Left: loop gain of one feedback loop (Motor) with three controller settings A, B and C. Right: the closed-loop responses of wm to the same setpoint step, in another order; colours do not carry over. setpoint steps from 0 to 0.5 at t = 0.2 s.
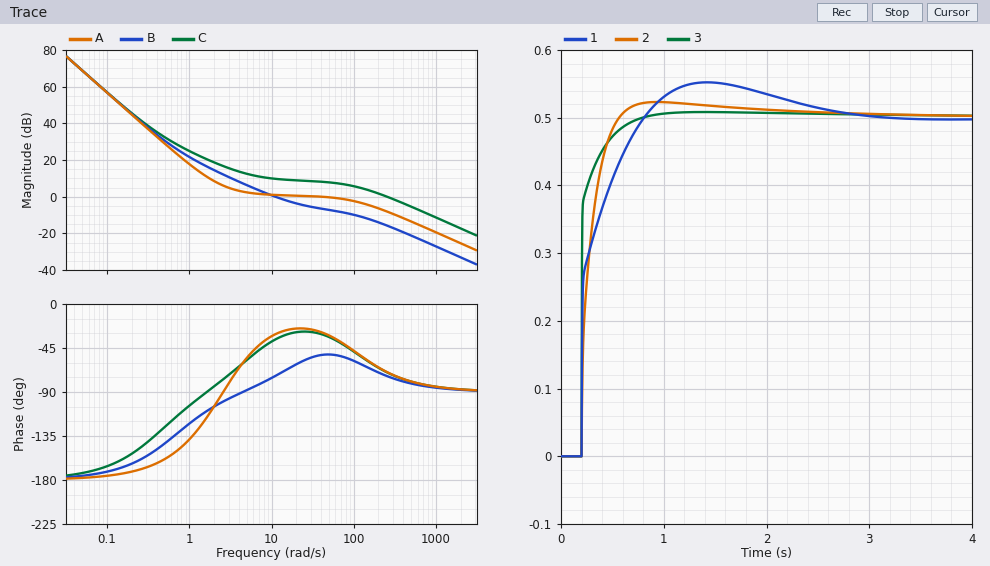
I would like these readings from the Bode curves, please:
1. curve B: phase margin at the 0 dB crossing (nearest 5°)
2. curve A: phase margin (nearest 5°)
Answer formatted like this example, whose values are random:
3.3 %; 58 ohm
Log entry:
105°; 150°
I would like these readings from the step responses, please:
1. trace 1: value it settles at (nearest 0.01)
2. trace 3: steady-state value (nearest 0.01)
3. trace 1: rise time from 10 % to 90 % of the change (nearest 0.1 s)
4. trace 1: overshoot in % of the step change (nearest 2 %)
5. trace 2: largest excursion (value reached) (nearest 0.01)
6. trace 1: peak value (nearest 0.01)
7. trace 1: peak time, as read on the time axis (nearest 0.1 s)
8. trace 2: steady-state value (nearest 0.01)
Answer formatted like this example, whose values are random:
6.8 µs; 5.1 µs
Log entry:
0.50; 0.50; 0.4 s; 10 %; 0.52; 0.55; 1.4 s; 0.50
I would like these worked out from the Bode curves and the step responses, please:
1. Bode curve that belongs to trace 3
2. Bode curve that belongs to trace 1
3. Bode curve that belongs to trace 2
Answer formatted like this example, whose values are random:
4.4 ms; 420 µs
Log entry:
C; A; B
